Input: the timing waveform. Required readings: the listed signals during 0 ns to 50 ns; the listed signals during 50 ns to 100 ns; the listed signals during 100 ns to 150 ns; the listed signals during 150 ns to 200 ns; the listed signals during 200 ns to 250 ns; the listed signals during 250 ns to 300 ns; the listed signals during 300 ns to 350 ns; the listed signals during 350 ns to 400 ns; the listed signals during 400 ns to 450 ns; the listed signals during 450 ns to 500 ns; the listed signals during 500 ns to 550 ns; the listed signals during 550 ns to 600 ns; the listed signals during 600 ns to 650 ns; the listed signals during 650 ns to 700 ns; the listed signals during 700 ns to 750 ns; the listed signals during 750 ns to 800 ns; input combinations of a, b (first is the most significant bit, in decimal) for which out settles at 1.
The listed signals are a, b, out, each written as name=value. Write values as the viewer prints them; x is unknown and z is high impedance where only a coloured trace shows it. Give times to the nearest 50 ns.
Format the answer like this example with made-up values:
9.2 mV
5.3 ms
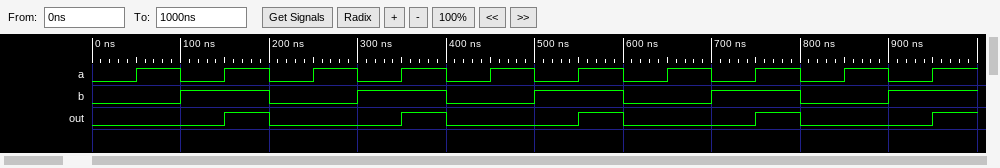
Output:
a=0, b=0, out=0
a=1, b=0, out=0
a=0, b=1, out=0
a=1, b=1, out=1
a=0, b=0, out=0
a=1, b=0, out=0
a=0, b=1, out=0
a=1, b=1, out=1
a=0, b=0, out=0
a=1, b=0, out=0
a=0, b=1, out=0
a=1, b=1, out=1
a=0, b=0, out=0
a=1, b=0, out=0
a=0, b=1, out=0
a=1, b=1, out=1
3
